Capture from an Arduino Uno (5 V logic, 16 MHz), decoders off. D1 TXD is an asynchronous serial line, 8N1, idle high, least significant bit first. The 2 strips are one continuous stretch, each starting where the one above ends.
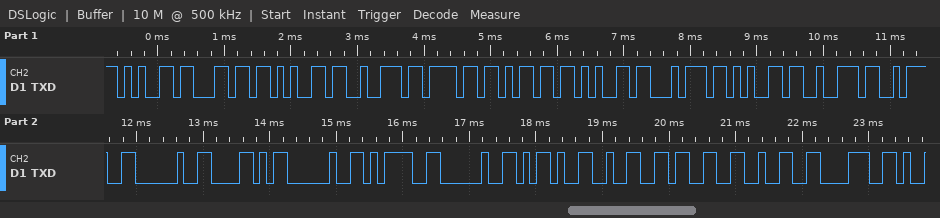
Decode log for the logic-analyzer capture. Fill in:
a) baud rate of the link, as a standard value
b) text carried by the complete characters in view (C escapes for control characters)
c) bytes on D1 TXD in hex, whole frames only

9600 baud
"elerometer: X = -2328"
0x65 0x6C 0x65 0x72 0x6F 0x6D 0x65 0x74 0x65 0x72 0x3A 0x20 0x58 0x20 0x3D 0x20 0x2D 0x32 0x33 0x32 0x38
